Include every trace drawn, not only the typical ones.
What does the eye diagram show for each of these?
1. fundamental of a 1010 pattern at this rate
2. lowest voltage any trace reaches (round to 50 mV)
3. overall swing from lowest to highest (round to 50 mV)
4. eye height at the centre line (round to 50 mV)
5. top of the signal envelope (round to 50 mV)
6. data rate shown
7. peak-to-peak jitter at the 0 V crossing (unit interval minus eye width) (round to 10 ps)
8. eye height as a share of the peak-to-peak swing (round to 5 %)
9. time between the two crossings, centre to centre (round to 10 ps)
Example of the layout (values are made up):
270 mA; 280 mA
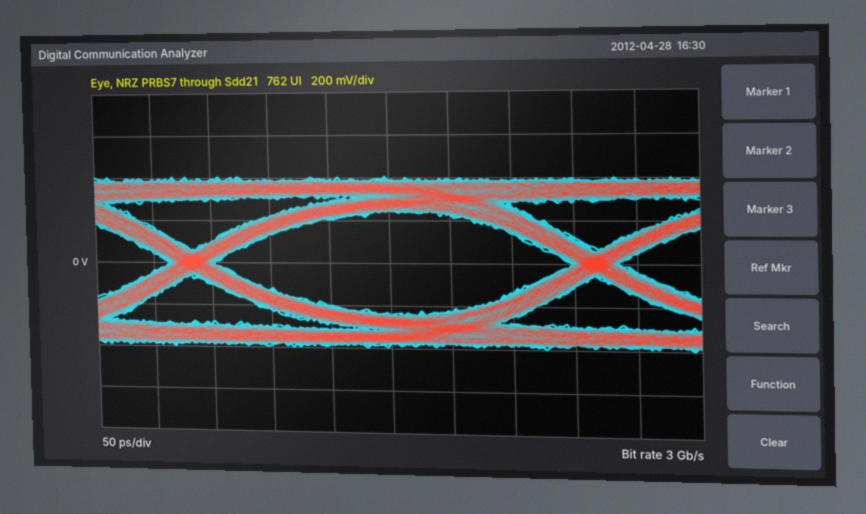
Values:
1.5 GHz; -400 mV; 800 mV; 500 mV; 400 mV; 3 Gb/s; 40 ps; 60 %; 330 ps
